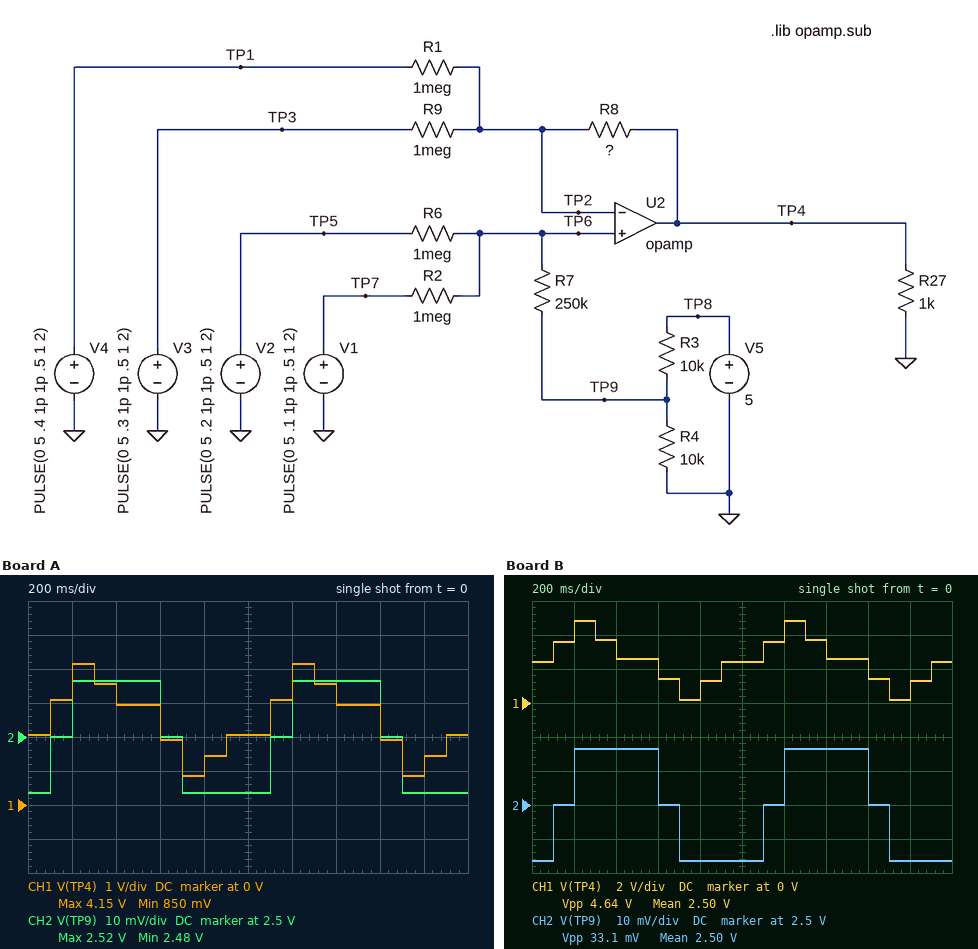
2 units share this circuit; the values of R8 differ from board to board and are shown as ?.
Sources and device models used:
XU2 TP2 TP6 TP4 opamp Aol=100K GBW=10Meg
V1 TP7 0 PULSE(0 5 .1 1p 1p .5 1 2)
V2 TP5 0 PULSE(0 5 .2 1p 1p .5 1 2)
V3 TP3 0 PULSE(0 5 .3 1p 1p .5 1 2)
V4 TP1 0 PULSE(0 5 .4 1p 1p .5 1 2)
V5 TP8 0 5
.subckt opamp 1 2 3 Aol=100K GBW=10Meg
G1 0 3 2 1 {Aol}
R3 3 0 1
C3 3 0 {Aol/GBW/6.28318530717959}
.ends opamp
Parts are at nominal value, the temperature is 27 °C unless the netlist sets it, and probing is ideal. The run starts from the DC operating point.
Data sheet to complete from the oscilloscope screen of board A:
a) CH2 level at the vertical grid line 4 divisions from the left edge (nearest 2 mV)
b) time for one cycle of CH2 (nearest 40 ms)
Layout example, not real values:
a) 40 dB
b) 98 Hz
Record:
a) 2.484 V
b) 1.00 s
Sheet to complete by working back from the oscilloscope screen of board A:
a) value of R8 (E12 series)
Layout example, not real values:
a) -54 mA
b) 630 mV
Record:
a) 120 kΩ
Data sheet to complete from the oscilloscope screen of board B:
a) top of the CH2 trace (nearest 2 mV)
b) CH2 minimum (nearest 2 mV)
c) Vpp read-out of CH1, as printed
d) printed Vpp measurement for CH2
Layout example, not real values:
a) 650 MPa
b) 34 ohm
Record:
a) 2.516 V
b) 2.484 V
c) 4.64 V
d) 33.1 mV
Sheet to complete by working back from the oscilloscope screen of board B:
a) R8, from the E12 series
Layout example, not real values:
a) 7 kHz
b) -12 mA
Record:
a) 220 kΩ
